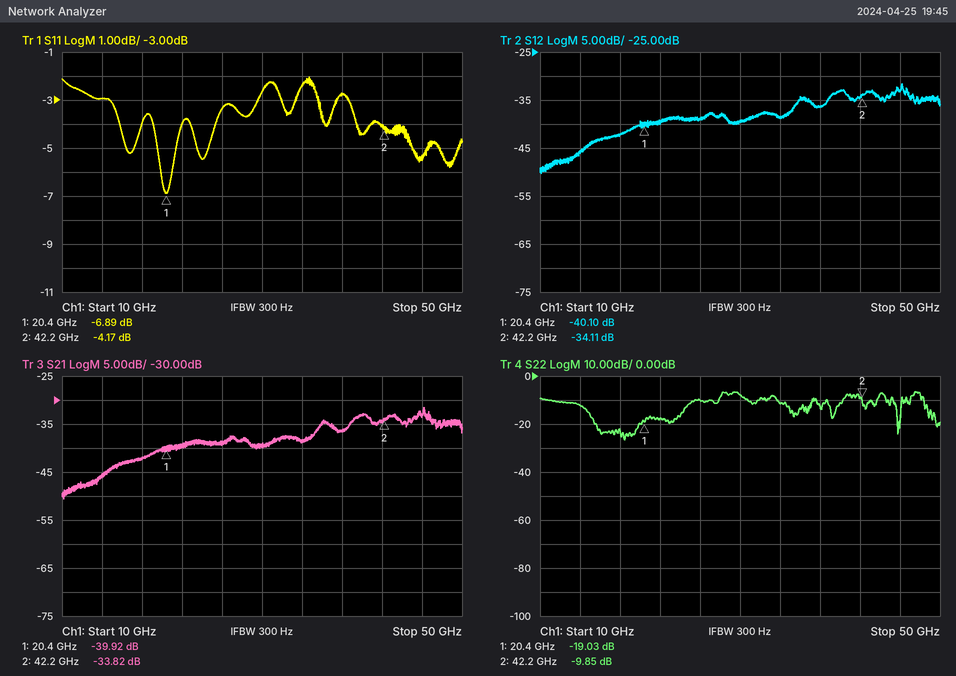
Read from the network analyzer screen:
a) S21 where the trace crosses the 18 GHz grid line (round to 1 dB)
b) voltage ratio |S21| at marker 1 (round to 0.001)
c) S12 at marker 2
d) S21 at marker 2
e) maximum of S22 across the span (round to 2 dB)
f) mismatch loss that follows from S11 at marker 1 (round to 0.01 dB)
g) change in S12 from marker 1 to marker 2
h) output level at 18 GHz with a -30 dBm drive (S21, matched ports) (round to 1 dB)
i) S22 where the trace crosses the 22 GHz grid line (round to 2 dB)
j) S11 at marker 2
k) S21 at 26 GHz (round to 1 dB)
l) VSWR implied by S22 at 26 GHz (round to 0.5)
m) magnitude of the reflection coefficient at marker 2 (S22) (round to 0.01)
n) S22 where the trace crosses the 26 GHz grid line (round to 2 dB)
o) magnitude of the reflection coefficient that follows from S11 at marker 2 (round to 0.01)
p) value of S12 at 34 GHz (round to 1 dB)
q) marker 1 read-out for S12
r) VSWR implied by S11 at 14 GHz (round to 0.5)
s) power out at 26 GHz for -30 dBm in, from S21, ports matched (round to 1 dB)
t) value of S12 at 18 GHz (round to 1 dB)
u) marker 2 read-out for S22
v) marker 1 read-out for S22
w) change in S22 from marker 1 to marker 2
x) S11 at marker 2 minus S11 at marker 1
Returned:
-42 dB
0.010
-34.11 dB
-33.82 dB
-6 dB
0.99 dB
5.99 dB
-72 dBm
-18 dB
-4.17 dB
-39 dB
2.0
0.32
-10 dB
0.62
-39 dB
-40.10 dB
6.0
-69 dBm
-42 dB
-9.85 dB
-19.03 dB
9.18 dB
2.72 dB
